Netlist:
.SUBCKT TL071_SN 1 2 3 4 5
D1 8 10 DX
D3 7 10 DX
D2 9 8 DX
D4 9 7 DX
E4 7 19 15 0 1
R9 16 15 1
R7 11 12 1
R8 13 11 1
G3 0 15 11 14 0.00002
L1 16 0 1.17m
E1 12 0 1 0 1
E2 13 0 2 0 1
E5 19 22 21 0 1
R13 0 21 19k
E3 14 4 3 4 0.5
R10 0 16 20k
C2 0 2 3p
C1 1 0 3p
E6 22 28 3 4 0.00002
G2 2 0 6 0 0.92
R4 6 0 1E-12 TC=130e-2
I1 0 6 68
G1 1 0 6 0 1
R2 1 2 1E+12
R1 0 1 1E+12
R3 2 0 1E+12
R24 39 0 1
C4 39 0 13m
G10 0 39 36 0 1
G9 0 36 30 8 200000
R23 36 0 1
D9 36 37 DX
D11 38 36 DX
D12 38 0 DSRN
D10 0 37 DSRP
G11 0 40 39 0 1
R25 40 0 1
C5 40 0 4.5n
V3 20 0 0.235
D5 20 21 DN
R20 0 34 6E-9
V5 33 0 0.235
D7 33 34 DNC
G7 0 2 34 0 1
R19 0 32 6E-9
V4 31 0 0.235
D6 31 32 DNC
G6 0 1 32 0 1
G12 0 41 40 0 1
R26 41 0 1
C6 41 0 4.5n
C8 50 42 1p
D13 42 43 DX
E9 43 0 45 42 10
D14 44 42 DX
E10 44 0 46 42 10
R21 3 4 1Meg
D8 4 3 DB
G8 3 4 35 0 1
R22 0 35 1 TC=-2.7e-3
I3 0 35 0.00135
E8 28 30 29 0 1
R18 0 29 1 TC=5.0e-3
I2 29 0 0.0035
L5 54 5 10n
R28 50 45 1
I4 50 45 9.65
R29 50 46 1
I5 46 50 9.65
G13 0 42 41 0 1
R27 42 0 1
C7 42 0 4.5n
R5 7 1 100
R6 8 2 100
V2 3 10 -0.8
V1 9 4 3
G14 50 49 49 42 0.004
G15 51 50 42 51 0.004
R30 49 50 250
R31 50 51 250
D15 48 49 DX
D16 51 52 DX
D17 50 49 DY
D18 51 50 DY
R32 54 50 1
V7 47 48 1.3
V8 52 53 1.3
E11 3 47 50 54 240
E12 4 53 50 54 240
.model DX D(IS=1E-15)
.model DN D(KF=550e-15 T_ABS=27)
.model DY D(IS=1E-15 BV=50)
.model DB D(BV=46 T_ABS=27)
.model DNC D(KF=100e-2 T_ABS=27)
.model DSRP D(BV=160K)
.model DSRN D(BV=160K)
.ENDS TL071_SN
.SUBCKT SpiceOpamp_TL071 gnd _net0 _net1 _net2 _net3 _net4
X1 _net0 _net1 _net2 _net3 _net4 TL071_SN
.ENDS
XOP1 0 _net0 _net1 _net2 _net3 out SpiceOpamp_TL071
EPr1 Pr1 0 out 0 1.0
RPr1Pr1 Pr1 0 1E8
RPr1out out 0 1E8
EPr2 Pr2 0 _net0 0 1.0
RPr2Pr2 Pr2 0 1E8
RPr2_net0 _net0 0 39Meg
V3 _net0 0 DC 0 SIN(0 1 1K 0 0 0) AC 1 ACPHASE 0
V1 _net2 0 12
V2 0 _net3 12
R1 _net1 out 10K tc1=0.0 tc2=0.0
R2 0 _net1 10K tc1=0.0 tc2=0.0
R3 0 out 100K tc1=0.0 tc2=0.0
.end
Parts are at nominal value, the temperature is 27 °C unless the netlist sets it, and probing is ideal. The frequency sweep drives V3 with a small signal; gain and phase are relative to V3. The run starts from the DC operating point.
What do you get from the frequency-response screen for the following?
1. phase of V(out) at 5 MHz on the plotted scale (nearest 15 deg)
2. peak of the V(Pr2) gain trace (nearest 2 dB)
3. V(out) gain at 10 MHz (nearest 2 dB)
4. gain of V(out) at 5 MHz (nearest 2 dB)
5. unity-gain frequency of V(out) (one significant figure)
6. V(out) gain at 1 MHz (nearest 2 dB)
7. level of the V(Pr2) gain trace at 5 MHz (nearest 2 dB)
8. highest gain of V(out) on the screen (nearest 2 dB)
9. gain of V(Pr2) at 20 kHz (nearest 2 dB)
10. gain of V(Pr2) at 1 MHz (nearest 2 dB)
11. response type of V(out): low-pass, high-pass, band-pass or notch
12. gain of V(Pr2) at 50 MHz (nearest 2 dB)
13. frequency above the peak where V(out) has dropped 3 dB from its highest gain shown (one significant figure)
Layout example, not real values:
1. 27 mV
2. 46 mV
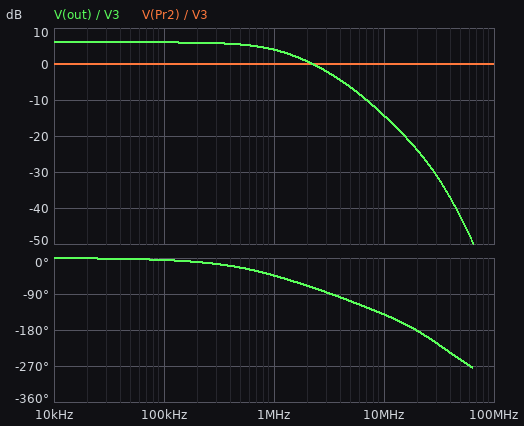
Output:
1. -105 deg
2. 0 dB
3. -14 dB
4. -6 dB
5. 2 MHz
6. 4 dB
7. 0 dB
8. 6 dB
9. 0 dB
10. 0 dB
11. low-pass
12. 0 dB
13. 1 MHz
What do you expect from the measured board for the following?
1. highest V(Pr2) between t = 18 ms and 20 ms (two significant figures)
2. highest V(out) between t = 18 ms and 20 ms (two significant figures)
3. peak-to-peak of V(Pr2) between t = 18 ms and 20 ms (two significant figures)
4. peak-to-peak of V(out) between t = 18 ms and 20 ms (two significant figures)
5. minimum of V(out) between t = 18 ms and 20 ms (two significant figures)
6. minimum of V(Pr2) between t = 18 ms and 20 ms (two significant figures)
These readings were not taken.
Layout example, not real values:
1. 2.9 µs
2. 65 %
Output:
1. 1.0 V
2. 2.0 V
3. 2.0 V
4. 4.0 V
5. -2.0 V
6. -1.0 V
